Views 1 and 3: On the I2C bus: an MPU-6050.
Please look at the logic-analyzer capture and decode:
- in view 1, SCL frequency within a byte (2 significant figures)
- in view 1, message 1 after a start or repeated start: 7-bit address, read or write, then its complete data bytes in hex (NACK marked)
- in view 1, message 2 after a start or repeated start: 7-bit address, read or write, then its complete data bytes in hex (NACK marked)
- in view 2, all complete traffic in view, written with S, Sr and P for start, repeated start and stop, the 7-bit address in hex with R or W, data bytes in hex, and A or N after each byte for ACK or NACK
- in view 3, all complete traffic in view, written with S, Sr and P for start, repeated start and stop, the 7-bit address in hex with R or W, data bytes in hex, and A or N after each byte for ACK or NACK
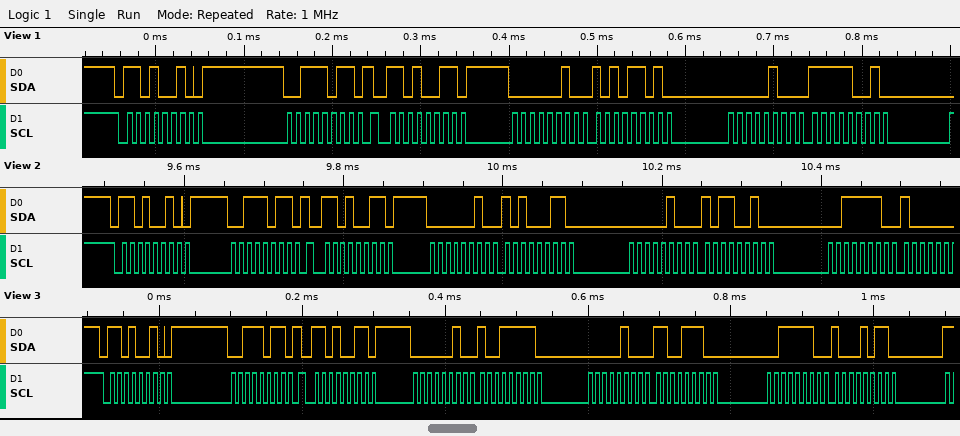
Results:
100 kHz
0x69 write: 3B
0x69 read: 02 AD 04 F9
S 69W A 3B A Sr 69R A 02 A A3 A 04 A B2 A 3E A
S 69W A 3B A Sr 69R A 02 A 9F A 04 A CE A 3E A 8B A
